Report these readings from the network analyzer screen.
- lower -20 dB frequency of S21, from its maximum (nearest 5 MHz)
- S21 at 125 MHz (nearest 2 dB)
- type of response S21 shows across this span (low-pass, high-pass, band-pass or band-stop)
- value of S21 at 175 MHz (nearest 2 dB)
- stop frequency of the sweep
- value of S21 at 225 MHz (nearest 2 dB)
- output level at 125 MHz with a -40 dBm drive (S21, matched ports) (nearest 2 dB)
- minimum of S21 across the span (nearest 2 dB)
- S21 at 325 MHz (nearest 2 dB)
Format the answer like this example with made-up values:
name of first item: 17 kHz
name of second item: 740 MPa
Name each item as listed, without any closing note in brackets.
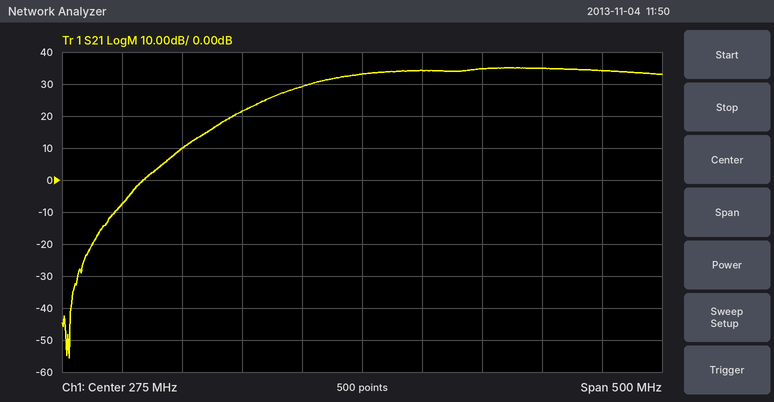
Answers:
lower -20 dB frequency of S21, from its maximum: 145 MHz
S21 at 125 MHz: 10 dB
type of response S21 shows across this span: high-pass
value of S21 at 175 MHz: 22 dB
stop frequency of the sweep: 525 MHz
value of S21 at 225 MHz: 30 dB
output level at 125 MHz with a -40 dBm drive (S21, matched ports): -30 dBm
minimum of S21 across the span: -56 dB
S21 at 325 MHz: 34 dB
